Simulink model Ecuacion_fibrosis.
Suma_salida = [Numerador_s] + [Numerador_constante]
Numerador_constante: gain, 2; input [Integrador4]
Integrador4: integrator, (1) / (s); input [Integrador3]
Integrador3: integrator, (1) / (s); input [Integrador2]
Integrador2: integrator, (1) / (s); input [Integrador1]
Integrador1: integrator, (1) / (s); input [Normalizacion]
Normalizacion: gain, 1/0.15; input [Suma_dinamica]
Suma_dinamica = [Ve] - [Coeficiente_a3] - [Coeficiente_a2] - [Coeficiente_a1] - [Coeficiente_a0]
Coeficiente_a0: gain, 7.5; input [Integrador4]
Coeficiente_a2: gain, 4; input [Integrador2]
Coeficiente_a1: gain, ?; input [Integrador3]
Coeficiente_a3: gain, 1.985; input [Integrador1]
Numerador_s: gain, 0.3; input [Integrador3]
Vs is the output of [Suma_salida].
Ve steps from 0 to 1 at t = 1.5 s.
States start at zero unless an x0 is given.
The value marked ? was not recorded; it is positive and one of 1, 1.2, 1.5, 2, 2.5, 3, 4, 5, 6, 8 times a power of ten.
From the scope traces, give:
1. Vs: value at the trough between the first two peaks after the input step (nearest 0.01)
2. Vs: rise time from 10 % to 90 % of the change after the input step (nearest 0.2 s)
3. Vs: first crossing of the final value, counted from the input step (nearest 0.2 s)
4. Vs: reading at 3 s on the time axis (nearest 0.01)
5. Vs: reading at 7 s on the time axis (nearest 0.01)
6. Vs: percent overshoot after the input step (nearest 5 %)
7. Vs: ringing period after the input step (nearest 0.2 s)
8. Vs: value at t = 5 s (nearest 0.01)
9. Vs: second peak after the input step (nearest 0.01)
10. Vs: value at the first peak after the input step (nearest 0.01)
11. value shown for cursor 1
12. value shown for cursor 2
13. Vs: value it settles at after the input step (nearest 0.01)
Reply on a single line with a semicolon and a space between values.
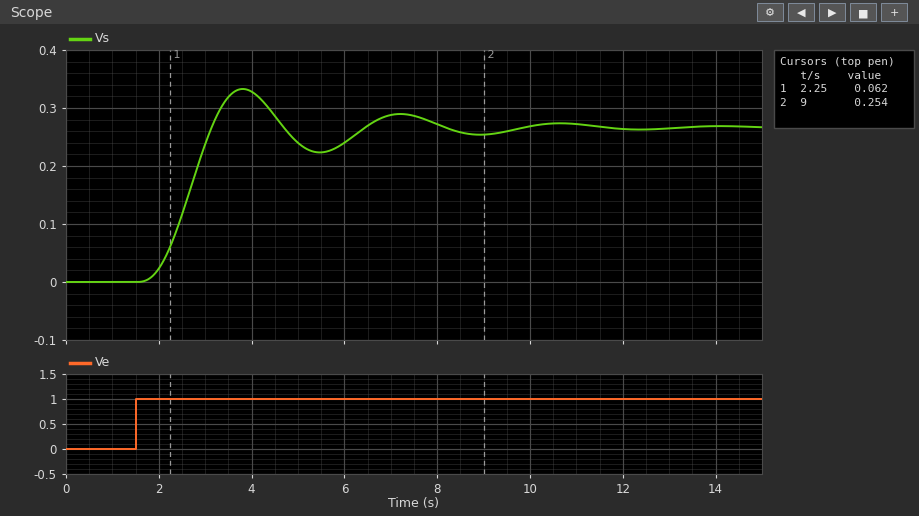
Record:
0.22; 1.0 s; 1.6 s; 0.24; 0.29; 25 %; 3.4 s; 0.24; 0.29; 0.33; 0.062; 0.254; 0.27
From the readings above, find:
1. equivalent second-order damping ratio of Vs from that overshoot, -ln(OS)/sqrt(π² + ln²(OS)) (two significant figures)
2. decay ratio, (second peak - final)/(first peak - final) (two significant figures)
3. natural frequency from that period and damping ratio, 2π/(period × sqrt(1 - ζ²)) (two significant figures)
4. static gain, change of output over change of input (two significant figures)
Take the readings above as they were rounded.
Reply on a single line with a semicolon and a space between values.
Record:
0.40; 0.33; 2.0 rad/s; 0.27
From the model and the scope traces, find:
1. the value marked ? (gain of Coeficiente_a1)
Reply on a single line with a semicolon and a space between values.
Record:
8
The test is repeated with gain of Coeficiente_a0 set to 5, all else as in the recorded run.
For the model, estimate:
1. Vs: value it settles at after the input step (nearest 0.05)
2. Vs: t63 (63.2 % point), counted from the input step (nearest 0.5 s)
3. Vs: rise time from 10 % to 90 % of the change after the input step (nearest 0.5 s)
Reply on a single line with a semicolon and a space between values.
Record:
0.40; 1.5 s; 1.5 s
